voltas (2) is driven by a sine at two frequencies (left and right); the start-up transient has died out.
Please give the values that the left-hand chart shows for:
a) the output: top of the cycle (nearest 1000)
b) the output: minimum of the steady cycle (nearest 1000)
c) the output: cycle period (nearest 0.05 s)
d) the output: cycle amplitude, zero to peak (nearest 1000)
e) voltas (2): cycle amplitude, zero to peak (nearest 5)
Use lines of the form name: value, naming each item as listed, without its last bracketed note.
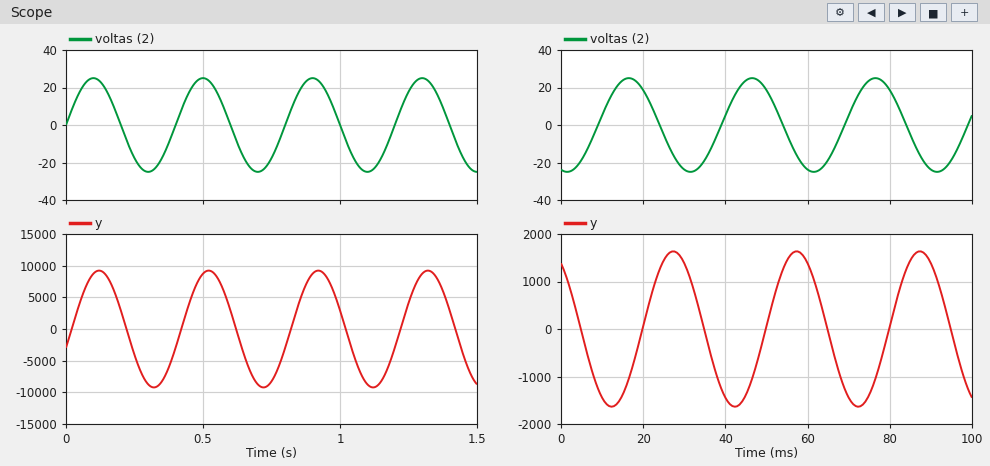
the output: top of the cycle: 9000
the output: minimum of the steady cycle: -9000
the output: cycle period: 0.40 s
the output: cycle amplitude, zero to peak: 9000
voltas (2): cycle amplitude, zero to peak: 25
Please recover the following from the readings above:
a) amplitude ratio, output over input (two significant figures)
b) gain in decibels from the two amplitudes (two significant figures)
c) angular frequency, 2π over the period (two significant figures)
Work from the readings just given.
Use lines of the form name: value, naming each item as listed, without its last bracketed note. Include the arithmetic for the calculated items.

amplitude ratio, output over input: 9000 / 25 = 360
gain in decibels from the two amplitudes: 20 log10(9000 / 25) = 51 dB
angular frequency, 2π over the period: 2π / 0.4 = 16 rad/s
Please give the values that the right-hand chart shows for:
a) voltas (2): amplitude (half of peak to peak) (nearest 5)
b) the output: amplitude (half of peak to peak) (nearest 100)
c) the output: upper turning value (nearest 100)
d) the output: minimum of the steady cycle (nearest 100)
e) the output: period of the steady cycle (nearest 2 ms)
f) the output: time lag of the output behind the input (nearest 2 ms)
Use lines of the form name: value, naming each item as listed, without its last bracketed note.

voltas (2): amplitude (half of peak to peak): 25
the output: amplitude (half of peak to peak): 1600
the output: upper turning value: 1600
the output: minimum of the steady cycle: -1600
the output: period of the steady cycle: 30 ms
the output: time lag of the output behind the input: 10 ms
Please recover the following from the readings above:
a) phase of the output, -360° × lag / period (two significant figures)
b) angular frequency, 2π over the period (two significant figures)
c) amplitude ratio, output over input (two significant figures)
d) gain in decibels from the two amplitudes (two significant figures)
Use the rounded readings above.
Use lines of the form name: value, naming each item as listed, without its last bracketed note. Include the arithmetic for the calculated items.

phase of the output, -360° × lag / period: -360 × 10 / 30 = -120°
angular frequency, 2π over the period: 2π / 30 = 0.21 rad/ms
amplitude ratio, output over input: 1600 / 25 = 64
gain in decibels from the two amplitudes: 20 log10(1600 / 25) = 36 dB
